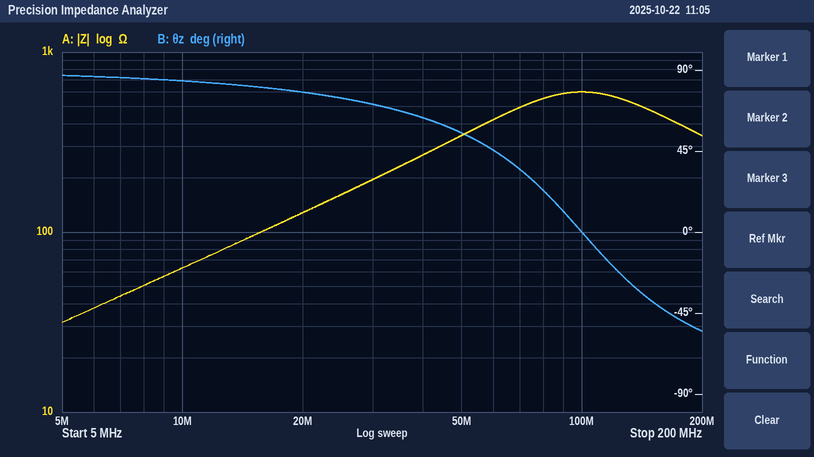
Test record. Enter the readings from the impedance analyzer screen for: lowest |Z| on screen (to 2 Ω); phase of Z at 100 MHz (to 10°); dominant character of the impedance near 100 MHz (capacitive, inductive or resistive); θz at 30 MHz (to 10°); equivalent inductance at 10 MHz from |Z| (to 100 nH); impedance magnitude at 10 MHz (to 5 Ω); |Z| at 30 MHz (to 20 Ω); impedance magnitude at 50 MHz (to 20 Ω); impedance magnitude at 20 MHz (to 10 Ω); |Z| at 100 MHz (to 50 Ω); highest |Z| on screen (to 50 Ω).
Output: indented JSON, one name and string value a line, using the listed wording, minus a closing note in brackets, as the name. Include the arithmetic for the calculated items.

{
  "lowest |Z| on screen": "32 Ω",
  "phase of Z at 100 MHz": "0°",
  "dominant character of the impedance near 100 MHz": "resistive",
  "θz at 30 MHz": "70°",
  "equivalent inductance at 10 MHz from |Z|": "L = 65 Ω/(2π × 10 MHz) ≈ 1.0 µH",
  "impedance magnitude at 10 MHz": "65 Ω",
  "|Z| at 30 MHz": "200 Ω",
  "impedance magnitude at 50 MHz": "340 Ω",
  "impedance magnitude at 20 MHz": "130 Ω",
  "|Z| at 100 MHz": "600 Ω",
  "highest |Z| on screen": "600 Ω"
}
